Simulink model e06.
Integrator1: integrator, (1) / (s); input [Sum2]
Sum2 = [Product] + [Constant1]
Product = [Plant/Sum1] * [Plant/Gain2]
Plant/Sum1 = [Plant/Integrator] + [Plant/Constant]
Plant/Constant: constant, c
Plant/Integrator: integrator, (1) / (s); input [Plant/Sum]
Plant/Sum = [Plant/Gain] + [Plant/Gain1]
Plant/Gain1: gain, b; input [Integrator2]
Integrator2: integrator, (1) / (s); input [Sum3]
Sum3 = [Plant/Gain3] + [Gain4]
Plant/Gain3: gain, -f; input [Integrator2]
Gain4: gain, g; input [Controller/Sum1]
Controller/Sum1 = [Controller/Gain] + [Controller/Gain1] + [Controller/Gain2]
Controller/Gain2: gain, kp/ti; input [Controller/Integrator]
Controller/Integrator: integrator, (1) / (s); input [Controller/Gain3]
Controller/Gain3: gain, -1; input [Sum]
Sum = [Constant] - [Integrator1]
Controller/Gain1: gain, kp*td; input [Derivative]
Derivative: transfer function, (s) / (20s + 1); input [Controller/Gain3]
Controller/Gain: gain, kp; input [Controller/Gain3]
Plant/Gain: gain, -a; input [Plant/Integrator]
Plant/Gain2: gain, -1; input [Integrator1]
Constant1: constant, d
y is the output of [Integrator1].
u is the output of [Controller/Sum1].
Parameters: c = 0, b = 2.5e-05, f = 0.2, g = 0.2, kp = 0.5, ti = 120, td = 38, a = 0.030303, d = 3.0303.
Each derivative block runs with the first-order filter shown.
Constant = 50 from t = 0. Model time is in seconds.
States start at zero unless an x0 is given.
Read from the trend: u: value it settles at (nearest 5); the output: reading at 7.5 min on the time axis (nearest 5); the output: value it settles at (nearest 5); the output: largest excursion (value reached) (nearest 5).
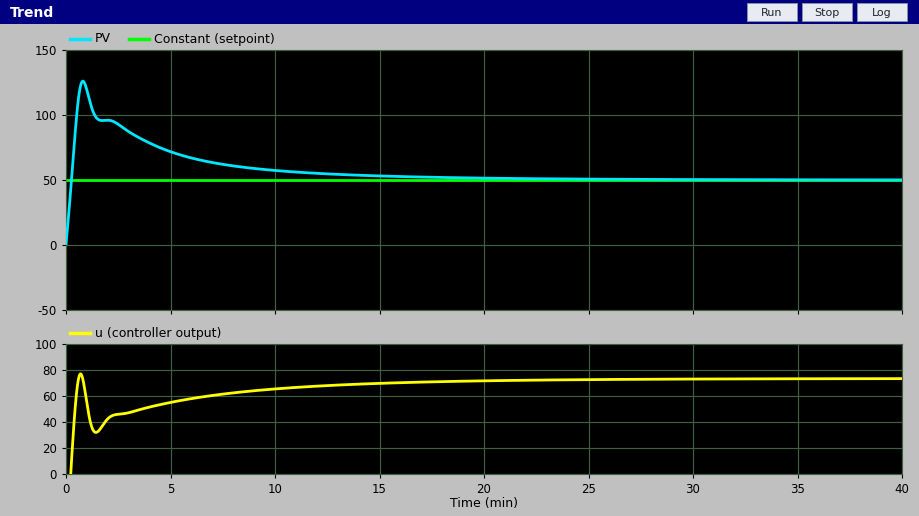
75
60
50
125
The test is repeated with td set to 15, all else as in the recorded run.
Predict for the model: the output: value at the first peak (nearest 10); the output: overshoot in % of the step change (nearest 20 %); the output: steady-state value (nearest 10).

140
180 %
50
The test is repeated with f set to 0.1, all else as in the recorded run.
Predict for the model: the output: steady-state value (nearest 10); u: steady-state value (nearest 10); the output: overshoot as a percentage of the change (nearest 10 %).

50
40
150 %
